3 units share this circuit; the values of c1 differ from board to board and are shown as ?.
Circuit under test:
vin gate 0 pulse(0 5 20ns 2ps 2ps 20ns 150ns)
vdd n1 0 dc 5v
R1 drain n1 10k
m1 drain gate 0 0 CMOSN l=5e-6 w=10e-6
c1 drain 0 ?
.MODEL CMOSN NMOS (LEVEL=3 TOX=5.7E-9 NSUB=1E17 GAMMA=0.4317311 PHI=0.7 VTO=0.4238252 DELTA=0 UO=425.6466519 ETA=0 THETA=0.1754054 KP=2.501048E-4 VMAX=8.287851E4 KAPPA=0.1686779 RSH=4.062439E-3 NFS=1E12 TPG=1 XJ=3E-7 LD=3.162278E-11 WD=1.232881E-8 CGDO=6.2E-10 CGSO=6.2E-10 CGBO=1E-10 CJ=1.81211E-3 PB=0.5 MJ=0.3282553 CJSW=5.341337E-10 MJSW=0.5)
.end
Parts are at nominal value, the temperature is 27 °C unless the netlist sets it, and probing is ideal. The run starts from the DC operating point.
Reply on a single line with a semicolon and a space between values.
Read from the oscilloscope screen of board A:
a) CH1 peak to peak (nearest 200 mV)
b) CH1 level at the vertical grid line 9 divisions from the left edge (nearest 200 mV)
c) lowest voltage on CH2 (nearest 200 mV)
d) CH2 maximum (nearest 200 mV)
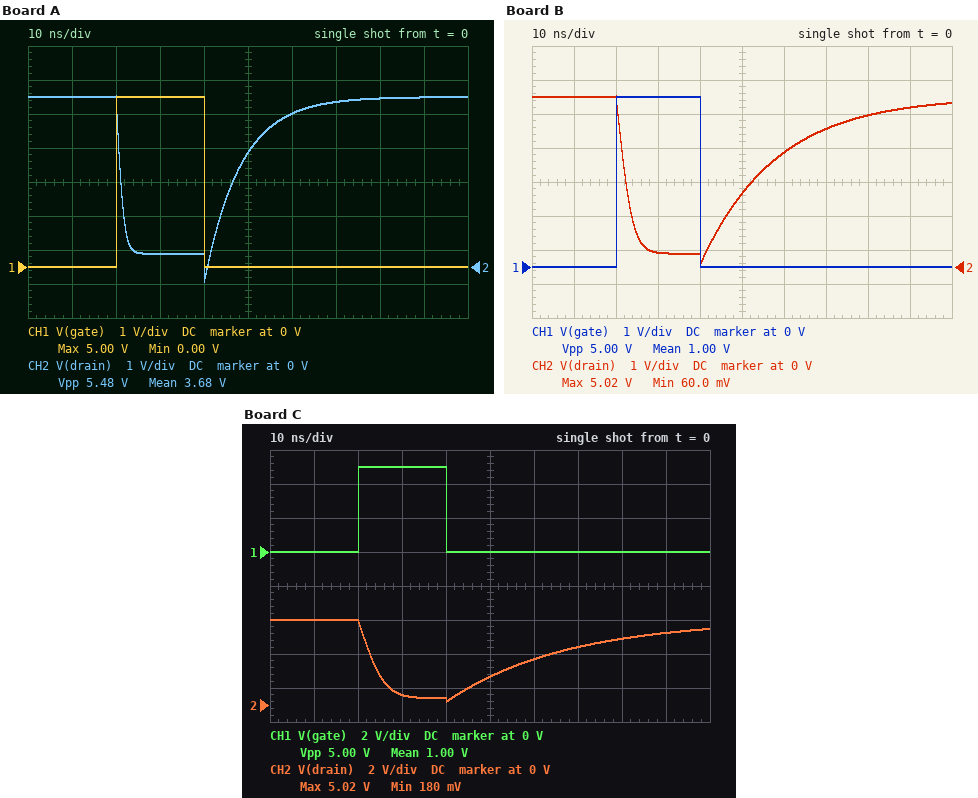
5.0 V; 0 V; -400 mV; 5.0 V
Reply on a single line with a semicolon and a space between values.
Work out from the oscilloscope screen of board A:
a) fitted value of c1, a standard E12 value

820 fF
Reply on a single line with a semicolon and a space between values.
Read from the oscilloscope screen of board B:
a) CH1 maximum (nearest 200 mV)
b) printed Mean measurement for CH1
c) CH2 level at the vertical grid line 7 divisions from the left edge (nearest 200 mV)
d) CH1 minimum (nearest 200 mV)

5.0 V; 1.00 V; 4.0 V; 0 V
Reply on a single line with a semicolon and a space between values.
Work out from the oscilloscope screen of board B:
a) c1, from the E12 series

1.8 pF
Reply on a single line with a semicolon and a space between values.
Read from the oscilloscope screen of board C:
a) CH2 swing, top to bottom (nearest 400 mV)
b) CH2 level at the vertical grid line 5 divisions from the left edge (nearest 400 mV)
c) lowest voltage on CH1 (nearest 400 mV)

4.8 V; 1.6 V; 0 V
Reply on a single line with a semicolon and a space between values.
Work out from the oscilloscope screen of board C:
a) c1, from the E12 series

2.7 pF
